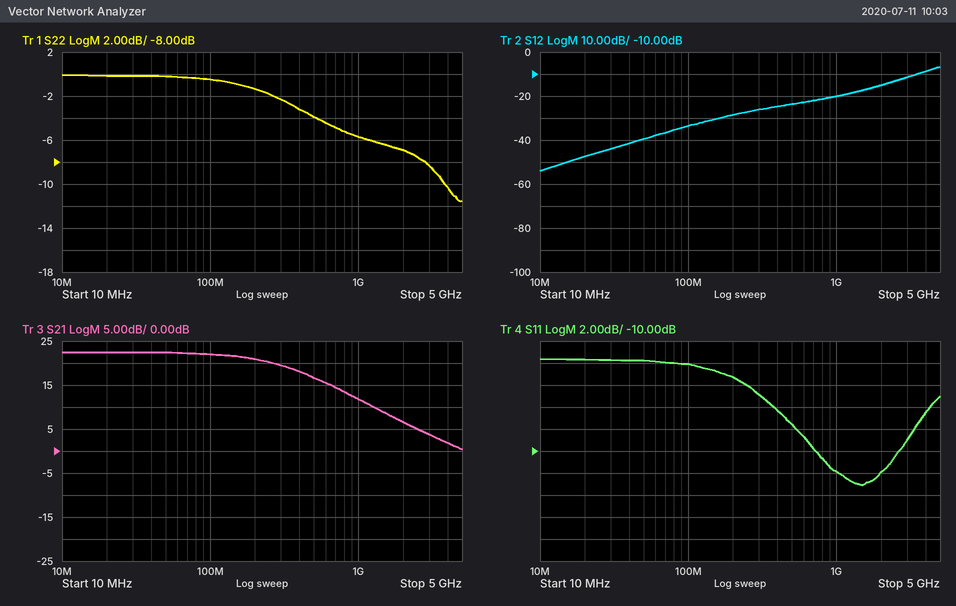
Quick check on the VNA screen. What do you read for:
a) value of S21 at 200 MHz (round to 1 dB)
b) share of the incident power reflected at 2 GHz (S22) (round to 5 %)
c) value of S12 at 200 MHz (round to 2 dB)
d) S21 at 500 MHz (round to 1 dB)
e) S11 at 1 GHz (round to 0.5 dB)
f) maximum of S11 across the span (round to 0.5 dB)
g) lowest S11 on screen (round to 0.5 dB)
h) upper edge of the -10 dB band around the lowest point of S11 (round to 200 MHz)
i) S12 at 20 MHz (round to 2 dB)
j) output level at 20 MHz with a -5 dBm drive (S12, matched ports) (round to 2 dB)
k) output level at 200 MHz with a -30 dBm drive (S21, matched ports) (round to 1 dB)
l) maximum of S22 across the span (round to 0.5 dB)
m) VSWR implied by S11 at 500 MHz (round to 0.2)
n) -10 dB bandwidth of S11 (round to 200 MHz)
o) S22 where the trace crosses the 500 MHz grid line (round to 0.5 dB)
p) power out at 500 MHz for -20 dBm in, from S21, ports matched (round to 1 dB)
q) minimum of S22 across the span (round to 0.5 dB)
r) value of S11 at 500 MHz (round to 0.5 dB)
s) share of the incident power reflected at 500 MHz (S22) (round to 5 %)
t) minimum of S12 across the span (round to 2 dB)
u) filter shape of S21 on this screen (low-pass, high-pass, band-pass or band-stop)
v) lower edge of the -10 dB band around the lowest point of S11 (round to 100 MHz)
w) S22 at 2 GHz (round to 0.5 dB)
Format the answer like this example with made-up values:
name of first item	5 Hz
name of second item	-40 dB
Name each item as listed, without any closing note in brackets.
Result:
value of S21 at 200 MHz	21 dB
share of the incident power reflected at 2 GHz (S22)	20 %
value of S12 at 200 MHz	-28 dB
S21 at 500 MHz	17 dB
S11 at 1 GHz	-12.0 dB
maximum of S11 across the span	-1.5 dB
lowest S11 on screen	-13.0 dB
upper edge of the -10 dB band around the lowest point of S11	2.6 GHz
S12 at 20 MHz	-48 dB
output level at 20 MHz with a -5 dBm drive (S12, matched ports)	-52 dBm
output level at 200 MHz with a -30 dBm drive (S21, matched ports)	-9 dBm
maximum of S22 across the span	0.0 dB
VSWR implied by S11 at 500 MHz	2.4
-10 dB bandwidth of S11	2.0 GHz
S22 where the trace crosses the 500 MHz grid line	-4.0 dB
power out at 500 MHz for -20 dBm in, from S21, ports matched	-3 dBm
minimum of S22 across the span	-11.5 dB
value of S11 at 500 MHz	-7.5 dB
share of the incident power reflected at 500 MHz (S22)	40 %
minimum of S12 across the span	-54 dB
filter shape of S21 on this screen	low-pass
lower edge of the -10 dB band around the lowest point of S11	700 MHz
S22 at 2 GHz	-7.0 dB
